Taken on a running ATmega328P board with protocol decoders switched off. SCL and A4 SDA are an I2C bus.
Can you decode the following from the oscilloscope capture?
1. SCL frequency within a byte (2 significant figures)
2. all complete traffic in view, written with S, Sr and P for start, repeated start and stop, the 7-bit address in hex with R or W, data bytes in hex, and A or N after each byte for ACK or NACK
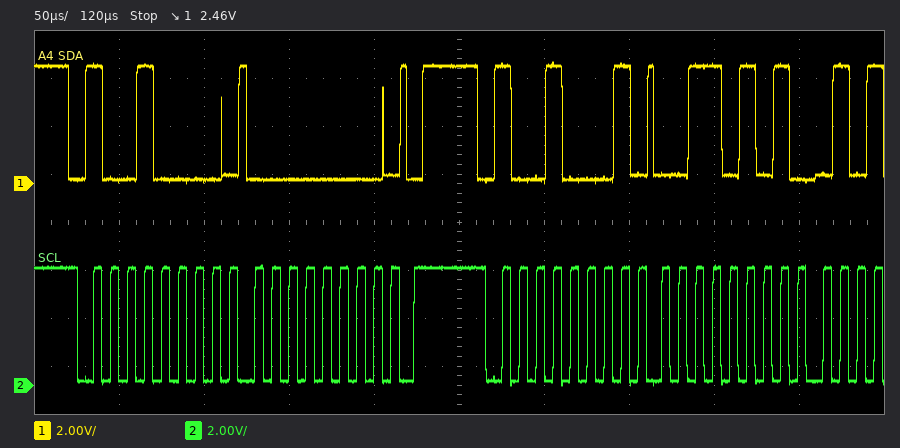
100 kHz
S 48W A 00 A P S 48R A 35 A
